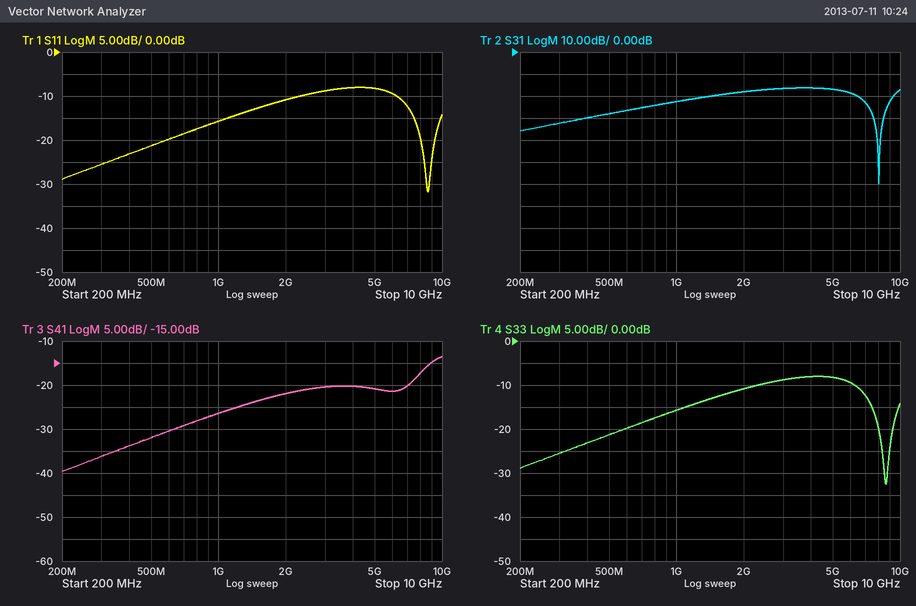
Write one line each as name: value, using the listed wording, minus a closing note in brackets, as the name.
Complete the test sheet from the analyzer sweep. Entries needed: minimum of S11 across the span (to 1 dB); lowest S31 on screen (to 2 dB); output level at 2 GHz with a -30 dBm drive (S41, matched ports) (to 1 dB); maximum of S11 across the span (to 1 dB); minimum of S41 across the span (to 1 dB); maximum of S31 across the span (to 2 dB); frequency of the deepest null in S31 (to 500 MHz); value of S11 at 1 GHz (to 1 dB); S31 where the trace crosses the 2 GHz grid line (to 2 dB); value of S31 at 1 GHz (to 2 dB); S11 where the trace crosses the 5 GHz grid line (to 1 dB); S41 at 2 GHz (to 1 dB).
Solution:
minimum of S11 across the span: -32 dB
lowest S31 on screen: -60 dB
output level at 2 GHz with a -30 dBm drive (S41, matched ports): -52 dBm
maximum of S11 across the span: -8 dB
minimum of S41 across the span: -40 dB
maximum of S31 across the span: -16 dB
frequency of the deepest null in S31: 8.0 GHz
value of S11 at 1 GHz: -16 dB
S31 where the trace crosses the 2 GHz grid line: -18 dB
value of S31 at 1 GHz: -22 dB
S11 where the trace crosses the 5 GHz grid line: -8 dB
S41 at 2 GHz: -22 dB
